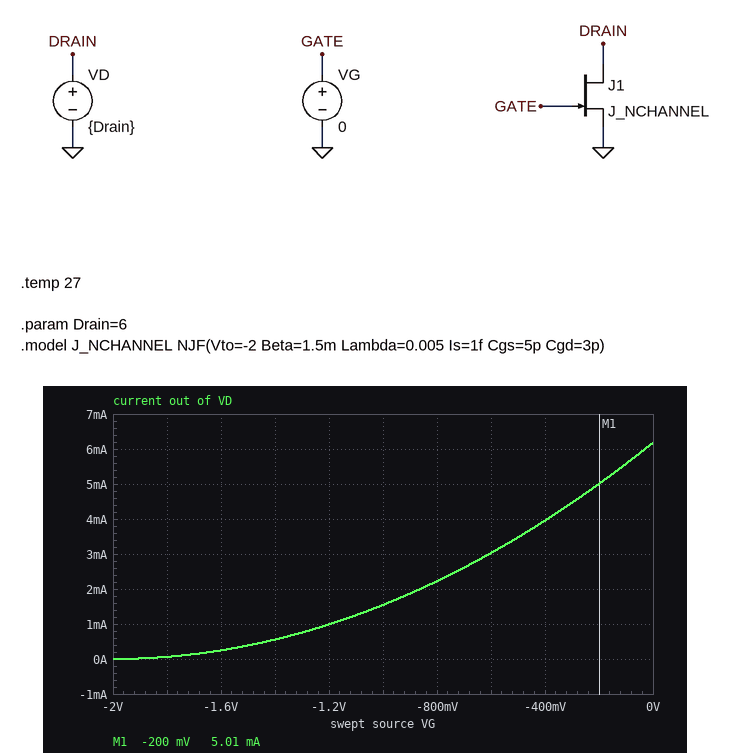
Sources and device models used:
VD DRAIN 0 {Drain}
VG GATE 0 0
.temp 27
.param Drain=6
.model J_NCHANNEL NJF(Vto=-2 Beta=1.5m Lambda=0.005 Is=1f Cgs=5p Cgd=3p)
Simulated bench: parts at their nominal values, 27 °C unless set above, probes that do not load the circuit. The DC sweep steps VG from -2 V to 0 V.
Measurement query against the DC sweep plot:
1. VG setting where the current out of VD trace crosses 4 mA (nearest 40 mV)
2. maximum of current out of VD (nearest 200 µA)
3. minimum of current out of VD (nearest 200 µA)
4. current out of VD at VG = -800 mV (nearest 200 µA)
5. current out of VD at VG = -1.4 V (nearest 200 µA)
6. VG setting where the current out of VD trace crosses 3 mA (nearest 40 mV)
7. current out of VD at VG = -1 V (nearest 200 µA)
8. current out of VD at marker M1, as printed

-400 mV
6.2 mA
0 A
2.2 mA
600 µA
-600 mV
1.6 mA
5.01 mA
